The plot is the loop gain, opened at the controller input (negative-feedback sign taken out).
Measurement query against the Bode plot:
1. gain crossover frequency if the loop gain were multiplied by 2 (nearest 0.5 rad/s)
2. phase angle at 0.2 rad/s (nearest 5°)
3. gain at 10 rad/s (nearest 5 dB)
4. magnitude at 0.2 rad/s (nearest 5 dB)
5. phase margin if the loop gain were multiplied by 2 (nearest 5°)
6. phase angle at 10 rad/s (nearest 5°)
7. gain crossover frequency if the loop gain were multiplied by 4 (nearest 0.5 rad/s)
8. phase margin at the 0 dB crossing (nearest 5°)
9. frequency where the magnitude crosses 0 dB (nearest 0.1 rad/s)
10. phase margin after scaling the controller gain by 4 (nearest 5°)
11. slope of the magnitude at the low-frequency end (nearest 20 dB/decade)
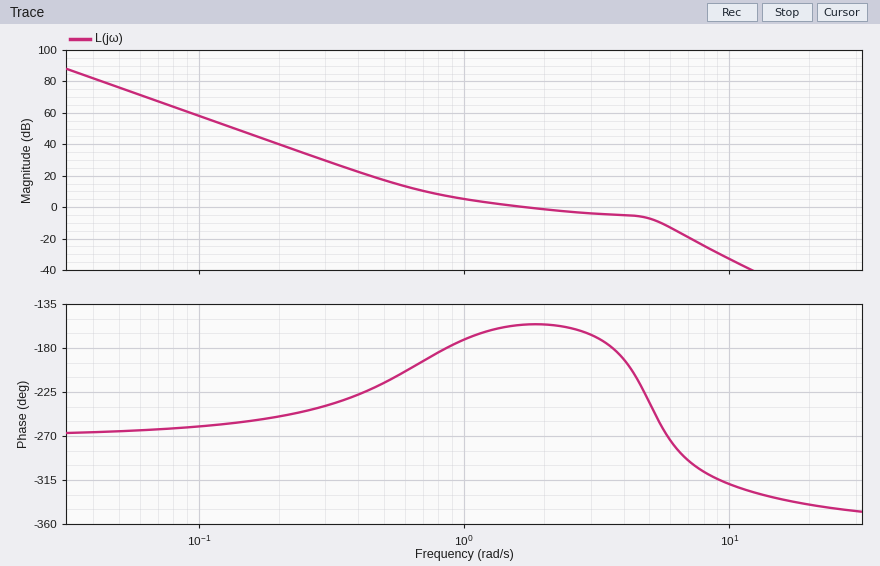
4.5 rad/s
-250°
-35 dB
40 dB
-40°
-320°
6.0 rad/s
25°
1.7 rad/s
-90°
-60 dB/decade
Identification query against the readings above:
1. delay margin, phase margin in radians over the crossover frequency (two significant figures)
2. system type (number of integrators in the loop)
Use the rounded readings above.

0.26 s
3
